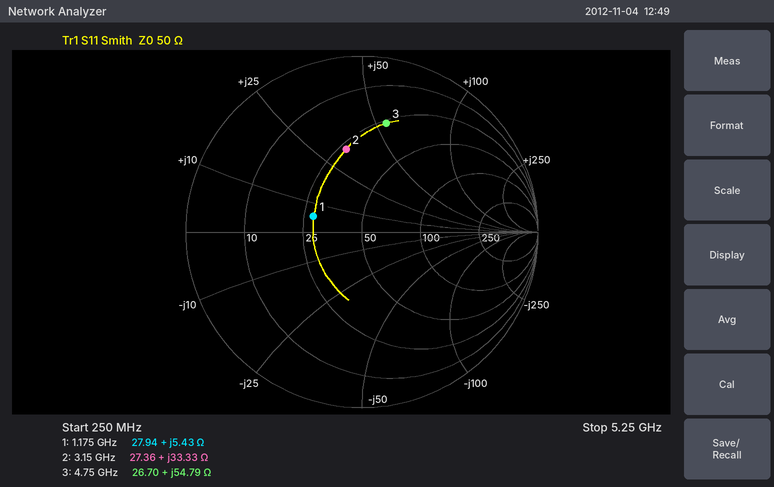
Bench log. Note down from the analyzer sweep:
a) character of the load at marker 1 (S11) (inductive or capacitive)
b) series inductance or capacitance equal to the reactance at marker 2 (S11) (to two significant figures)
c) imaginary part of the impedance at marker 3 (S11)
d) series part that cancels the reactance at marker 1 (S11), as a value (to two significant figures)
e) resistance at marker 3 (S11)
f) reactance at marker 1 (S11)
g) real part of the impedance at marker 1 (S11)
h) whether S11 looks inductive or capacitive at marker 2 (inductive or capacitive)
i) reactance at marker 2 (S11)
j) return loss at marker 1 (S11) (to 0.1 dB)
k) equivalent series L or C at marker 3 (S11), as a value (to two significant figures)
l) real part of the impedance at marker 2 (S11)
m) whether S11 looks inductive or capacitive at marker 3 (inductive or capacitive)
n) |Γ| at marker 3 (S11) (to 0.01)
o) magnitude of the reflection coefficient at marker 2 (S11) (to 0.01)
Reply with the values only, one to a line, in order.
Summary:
inductive
1.7 nH
+54.79 Ω
25 pF
26.70 Ω
+5.43 Ω
27.94 Ω
inductive
+33.33 Ω
10.7 dB
1.8 nH
27.36 Ω
inductive
0.63
0.48
